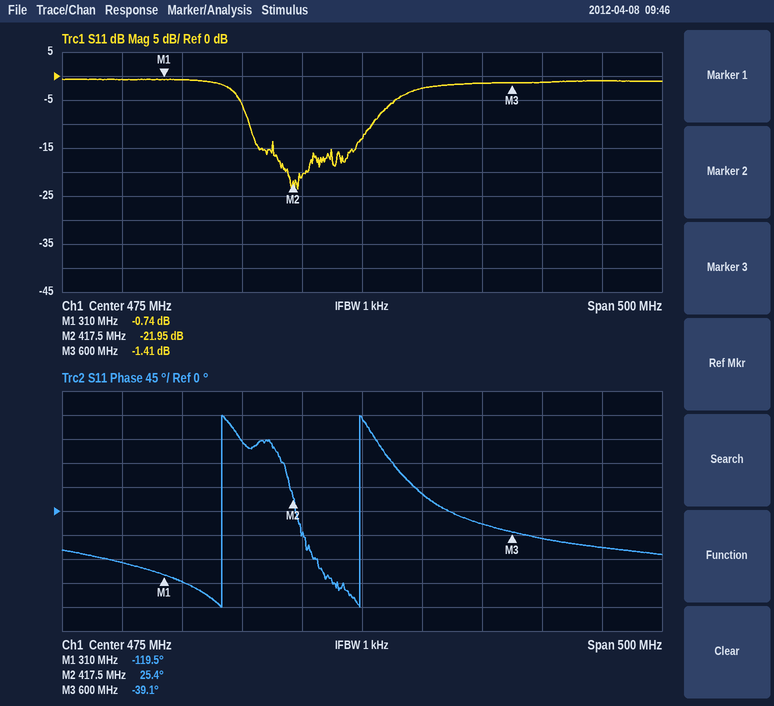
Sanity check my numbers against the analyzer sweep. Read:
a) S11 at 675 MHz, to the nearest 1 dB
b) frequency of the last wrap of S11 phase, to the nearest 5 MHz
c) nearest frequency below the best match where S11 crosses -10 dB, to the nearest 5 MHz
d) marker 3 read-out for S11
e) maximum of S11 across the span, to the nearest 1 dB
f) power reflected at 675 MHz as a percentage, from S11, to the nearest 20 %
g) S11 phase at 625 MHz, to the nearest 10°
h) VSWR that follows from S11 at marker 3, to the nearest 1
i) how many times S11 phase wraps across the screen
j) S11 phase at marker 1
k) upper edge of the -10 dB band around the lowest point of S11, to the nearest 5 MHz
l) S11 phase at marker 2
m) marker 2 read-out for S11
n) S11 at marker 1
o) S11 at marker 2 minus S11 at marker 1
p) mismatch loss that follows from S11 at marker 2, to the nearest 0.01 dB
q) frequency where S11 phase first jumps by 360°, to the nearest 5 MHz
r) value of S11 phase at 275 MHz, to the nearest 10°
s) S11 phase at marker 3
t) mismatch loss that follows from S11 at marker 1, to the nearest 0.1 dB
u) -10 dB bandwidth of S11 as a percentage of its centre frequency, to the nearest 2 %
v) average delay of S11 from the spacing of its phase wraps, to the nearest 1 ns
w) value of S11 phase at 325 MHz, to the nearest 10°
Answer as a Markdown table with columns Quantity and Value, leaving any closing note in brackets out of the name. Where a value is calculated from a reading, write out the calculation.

| Quantity | Value |
|---|---|
| S11 at 675 MHz, to the nearest 1 dB | -1 dB |
| frequency of the last wrap of S11 phase, to the nearest 5 MHz | 475 MHz |
| nearest frequency below the best match where S11 crosses -10 dB, to the nearest 5 MHz | 380 MHz |
| marker 3 read-out for S11 | -1.41 dB |
| maximum of S11 across the span, to the nearest 1 dB | -1 dB |
| power reflected at 675 MHz as a percentage, from S11, to the nearest 20 % | 10^(-1/10) ≈ 79.4 %, so 80 % to the nearest 20 % |
| S11 phase at 625 MHz, to the nearest 10° | -50° |
| VSWR that follows from S11 at marker 3, to the nearest 1 | (1 + 0.8502)/(1 − 0.8502) ≈ 12 |
| how many times S11 phase wraps across the screen | 2 |
| S11 phase at marker 1 | -119.5° |
| upper edge of the -10 dB band around the lowest point of S11, to the nearest 5 MHz | 485 MHz |
| S11 phase at marker 2 | 25.4° |
| marker 2 read-out for S11 | -21.95 dB |
| S11 at marker 1 | -0.74 dB |
| S11 at marker 2 minus S11 at marker 1 | -21.95 − (-0.74) = -21.21 dB |
| mismatch loss that follows from S11 at marker 2, to the nearest 0.01 dB | −10 log10(1 − 10^(-21.95/10)) ≈ 0.03 dB |
| frequency where S11 phase first jumps by 360°, to the nearest 5 MHz | 360 MHz |
| value of S11 phase at 275 MHz, to the nearest 10° | -100° |
| S11 phase at marker 3 | -39.1° |
| mismatch loss that follows from S11 at marker 1, to the nearest 0.1 dB | −10 log10(1 − 10^(-0.74/10)) ≈ 8.1 dB |
| -10 dB bandwidth of S11 as a percentage of its centre frequency, to the nearest 2 % | 105 MHz / 432.5 MHz ≈ 24 % |
| average delay of S11 from the spacing of its phase wraps, to the nearest 1 ns | 1 cycle / (475 MHz − 360 MHz) ≈ 9 ns |
| value of S11 phase at 325 MHz, to the nearest 10° | -130° |
